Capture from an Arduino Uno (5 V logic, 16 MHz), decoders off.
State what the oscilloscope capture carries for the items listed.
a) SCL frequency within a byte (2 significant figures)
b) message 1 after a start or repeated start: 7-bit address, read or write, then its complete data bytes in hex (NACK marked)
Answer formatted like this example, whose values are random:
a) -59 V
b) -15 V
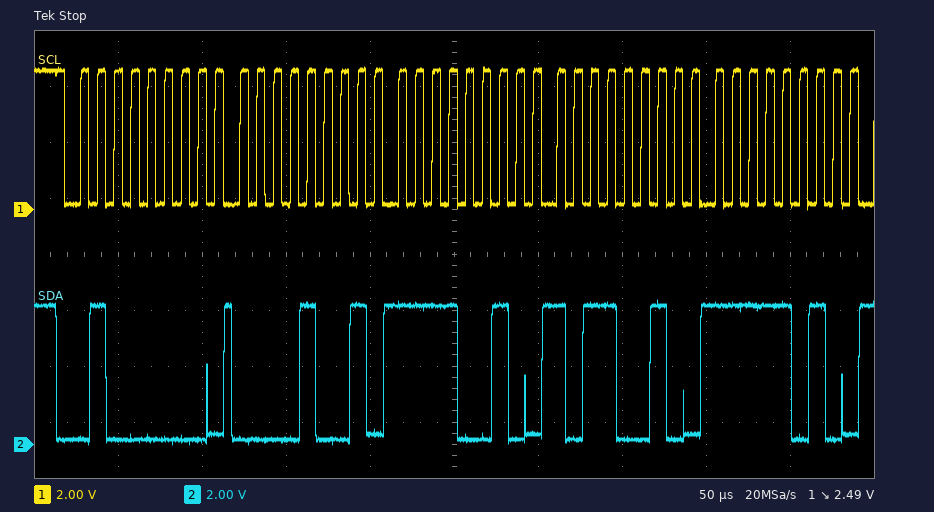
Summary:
a) 100 kHz
b) 0x20 write: 09 F2 B2 FA
